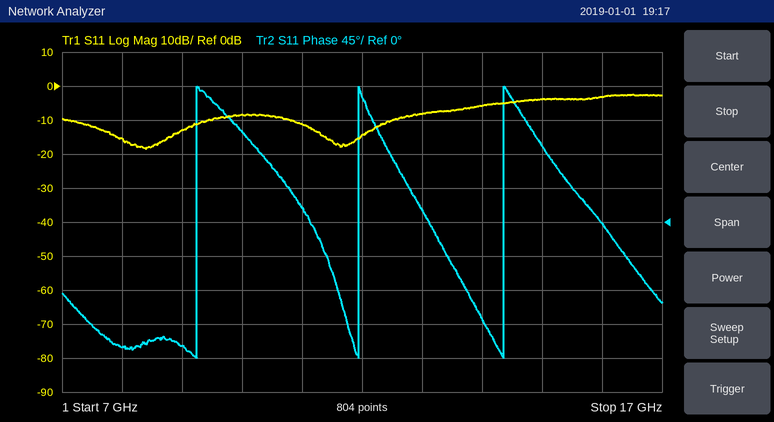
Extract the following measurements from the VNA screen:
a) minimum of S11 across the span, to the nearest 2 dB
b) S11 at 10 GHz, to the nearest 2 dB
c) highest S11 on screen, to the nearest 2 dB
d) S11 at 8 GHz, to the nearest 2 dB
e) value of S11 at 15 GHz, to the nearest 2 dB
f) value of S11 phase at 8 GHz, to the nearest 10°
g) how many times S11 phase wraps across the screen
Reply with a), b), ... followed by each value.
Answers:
a) -18 dB
b) -8 dB
c) -2 dB
d) -16 dB
e) -4 dB
f) -170°
g) 3
